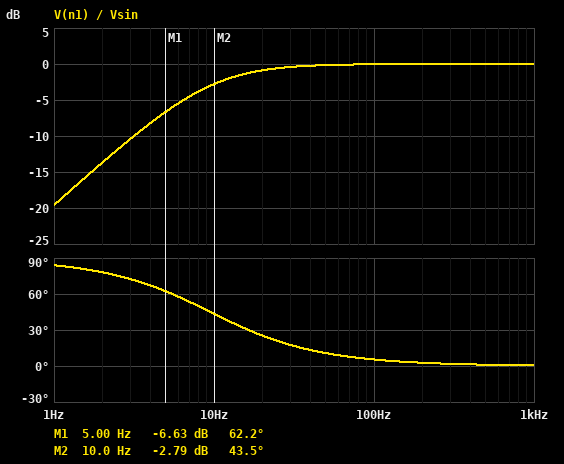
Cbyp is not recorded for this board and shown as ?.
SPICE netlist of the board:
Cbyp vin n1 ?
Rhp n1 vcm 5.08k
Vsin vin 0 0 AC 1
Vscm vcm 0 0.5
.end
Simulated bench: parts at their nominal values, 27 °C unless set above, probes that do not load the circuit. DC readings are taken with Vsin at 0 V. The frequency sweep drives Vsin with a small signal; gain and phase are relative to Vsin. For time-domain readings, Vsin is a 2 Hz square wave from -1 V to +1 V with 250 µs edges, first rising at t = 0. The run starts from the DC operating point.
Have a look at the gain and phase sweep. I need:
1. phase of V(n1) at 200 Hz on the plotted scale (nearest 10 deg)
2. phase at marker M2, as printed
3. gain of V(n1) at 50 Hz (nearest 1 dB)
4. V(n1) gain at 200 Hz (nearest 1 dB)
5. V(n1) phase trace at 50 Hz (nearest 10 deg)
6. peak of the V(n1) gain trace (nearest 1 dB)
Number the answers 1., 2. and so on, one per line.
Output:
1. 0 deg
2. 43.5 deg
3. 0 dB
4. 0 dB
5. 10 deg
6. 0 dB
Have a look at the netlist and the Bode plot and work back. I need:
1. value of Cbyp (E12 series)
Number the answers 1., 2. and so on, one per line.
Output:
1. 3.3 µF
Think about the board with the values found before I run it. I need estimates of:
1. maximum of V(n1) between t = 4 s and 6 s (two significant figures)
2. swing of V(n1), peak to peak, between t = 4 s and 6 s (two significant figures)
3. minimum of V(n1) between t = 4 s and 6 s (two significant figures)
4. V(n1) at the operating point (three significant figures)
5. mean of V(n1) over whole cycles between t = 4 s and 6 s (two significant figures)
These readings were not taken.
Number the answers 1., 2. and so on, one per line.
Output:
1. 2.5 V
2. 4.0 V
3. -1.5 V
4. 500 mV
5. 500 mV
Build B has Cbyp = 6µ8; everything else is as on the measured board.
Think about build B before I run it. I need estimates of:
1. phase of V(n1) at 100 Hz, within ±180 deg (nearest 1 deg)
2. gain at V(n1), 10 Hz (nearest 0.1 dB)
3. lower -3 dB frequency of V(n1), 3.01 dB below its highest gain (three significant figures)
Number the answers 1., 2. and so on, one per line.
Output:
1. 3 deg
2. -0.8 dB
3. 4.61 Hz
